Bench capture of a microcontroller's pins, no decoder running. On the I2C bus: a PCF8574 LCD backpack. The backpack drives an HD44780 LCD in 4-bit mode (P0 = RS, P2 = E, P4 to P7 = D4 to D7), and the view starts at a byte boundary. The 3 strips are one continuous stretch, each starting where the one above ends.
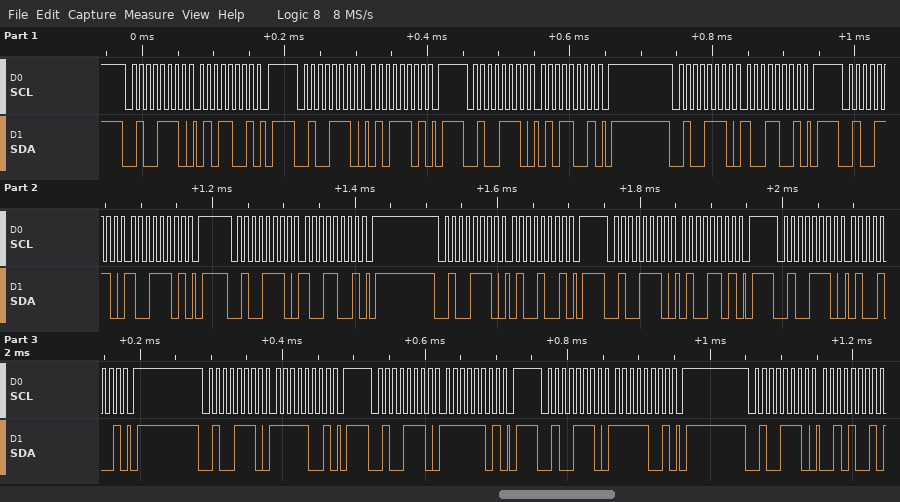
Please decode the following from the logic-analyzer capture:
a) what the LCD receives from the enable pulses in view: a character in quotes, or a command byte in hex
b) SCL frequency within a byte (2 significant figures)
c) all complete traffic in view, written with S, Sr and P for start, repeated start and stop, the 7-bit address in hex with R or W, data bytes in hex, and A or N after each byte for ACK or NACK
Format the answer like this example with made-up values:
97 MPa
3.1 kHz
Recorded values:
'Y' 'O'
100 kHz
S 27W A 59 A P S 27W A 5D A P S 27W A 59 A P S 27W A 99 A P S 27W A 9D A P S 27W A 99 A P S 27W A 49 A P S 27W A 4D A P S 27W A 49 A P S 27W A F9 A P S 27W A FD A P S 27W A F9 A P S 27W A 29 A
